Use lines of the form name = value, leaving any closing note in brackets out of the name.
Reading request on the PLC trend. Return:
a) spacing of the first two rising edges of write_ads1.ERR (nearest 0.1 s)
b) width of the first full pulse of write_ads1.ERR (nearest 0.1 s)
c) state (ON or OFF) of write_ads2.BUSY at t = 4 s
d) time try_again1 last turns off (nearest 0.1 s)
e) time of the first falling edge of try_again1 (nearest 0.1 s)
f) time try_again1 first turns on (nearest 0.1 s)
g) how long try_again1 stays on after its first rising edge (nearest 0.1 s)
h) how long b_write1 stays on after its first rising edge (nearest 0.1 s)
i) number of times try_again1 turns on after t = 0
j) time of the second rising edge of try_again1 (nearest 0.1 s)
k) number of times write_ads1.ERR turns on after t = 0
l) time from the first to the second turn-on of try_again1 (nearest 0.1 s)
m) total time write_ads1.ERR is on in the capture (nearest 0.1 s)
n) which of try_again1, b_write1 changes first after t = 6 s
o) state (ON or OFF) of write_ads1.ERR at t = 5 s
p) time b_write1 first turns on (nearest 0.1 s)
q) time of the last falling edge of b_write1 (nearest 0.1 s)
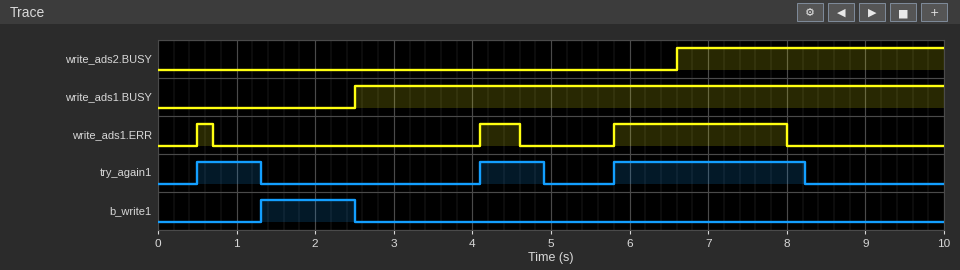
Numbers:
spacing of the first two rising edges of write_ads1.ERR = 3.6 s
width of the first full pulse of write_ads1.ERR = 0.2 s
state (ON or OFF) of write_ads2.BUSY at t = 4 s = OFF
time try_again1 last turns off = 8.2 s
time of the first falling edge of try_again1 = 1.3 s
time try_again1 first turns on = 0.5 s
how long try_again1 stays on after its first rising edge = 0.8 s
how long b_write1 stays on after its first rising edge = 1.2 s
number of times try_again1 turns on after t = 0 = 3
time of the second rising edge of try_again1 = 4.1 s
number of times write_ads1.ERR turns on after t = 0 = 3
time from the first to the second turn-on of try_again1 = 3.6 s
total time write_ads1.ERR is on in the capture = 2.9 s
which of try_again1, b_write1 changes first after t = 6 s = try_again1
state (ON or OFF) of write_ads1.ERR at t = 5 s = OFF
time b_write1 first turns on = 1.3 s
time of the last falling edge of b_write1 = 2.5 s
